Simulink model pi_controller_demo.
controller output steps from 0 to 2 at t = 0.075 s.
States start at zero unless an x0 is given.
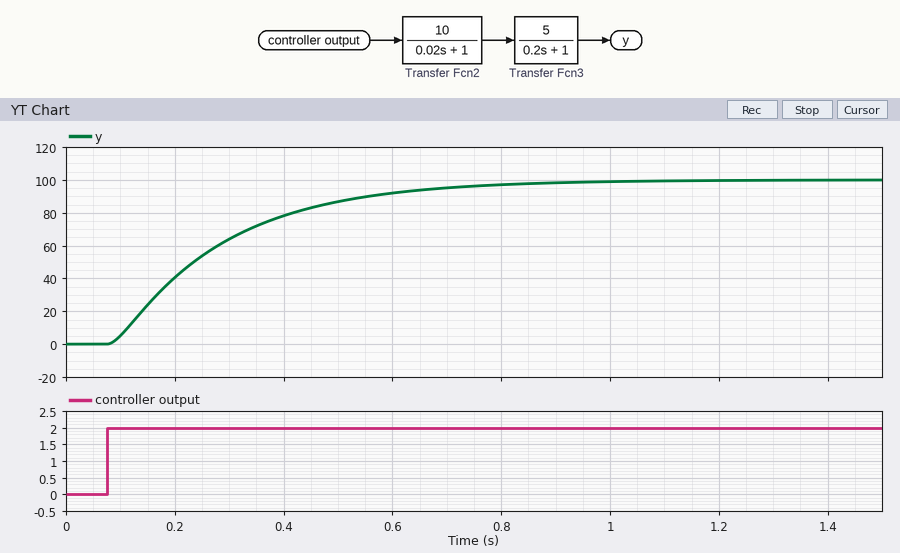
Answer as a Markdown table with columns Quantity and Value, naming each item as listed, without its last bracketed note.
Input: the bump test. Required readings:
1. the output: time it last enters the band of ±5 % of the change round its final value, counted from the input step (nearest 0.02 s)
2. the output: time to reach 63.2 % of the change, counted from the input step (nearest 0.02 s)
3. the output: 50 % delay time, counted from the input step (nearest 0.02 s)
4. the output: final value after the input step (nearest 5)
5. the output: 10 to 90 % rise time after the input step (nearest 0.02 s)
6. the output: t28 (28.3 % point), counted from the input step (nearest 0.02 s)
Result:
| Quantity | Value |
|---|---|
| the output: time it last enters the band of ±5 % of the change round its final value, counted from the input step | 0.62 s |
| the output: time to reach 63.2 % of the change, counted from the input step | 0.22 s |
| the output: 50 % delay time, counted from the input step | 0.16 s |
| the output: final value after the input step | 100 |
| the output: 10 to 90 % rise time after the input step | 0.44 s |
| the output: t28 (28.3 % point), counted from the input step | 0.08 s |
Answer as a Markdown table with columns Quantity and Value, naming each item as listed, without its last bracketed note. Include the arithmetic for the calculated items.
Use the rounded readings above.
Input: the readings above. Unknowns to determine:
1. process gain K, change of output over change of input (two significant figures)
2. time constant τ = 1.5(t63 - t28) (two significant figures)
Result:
| Quantity | Value |
|---|---|
| process gain K, change of output over change of input | (100 - 0) / 2 = 50 |
| time constant τ = 1.5(t63 - t28) | 1.5 × (0.22 - 0.08) = 0.21 s |
